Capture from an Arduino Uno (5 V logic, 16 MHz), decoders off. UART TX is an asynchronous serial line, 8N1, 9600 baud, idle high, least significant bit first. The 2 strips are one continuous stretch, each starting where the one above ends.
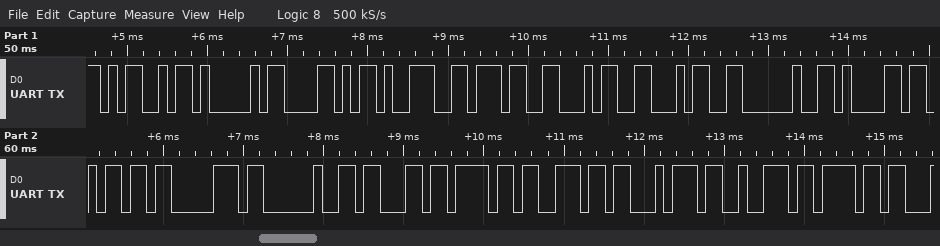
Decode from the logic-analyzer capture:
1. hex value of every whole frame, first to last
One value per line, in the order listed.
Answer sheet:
0x4D 0x41 0x58 0x39 0x37 0x34 0x34 0x20 0x61 0x6D 0x70 0x20 0x63 0x6F 0x6E 0x74 0x72 0x6F
